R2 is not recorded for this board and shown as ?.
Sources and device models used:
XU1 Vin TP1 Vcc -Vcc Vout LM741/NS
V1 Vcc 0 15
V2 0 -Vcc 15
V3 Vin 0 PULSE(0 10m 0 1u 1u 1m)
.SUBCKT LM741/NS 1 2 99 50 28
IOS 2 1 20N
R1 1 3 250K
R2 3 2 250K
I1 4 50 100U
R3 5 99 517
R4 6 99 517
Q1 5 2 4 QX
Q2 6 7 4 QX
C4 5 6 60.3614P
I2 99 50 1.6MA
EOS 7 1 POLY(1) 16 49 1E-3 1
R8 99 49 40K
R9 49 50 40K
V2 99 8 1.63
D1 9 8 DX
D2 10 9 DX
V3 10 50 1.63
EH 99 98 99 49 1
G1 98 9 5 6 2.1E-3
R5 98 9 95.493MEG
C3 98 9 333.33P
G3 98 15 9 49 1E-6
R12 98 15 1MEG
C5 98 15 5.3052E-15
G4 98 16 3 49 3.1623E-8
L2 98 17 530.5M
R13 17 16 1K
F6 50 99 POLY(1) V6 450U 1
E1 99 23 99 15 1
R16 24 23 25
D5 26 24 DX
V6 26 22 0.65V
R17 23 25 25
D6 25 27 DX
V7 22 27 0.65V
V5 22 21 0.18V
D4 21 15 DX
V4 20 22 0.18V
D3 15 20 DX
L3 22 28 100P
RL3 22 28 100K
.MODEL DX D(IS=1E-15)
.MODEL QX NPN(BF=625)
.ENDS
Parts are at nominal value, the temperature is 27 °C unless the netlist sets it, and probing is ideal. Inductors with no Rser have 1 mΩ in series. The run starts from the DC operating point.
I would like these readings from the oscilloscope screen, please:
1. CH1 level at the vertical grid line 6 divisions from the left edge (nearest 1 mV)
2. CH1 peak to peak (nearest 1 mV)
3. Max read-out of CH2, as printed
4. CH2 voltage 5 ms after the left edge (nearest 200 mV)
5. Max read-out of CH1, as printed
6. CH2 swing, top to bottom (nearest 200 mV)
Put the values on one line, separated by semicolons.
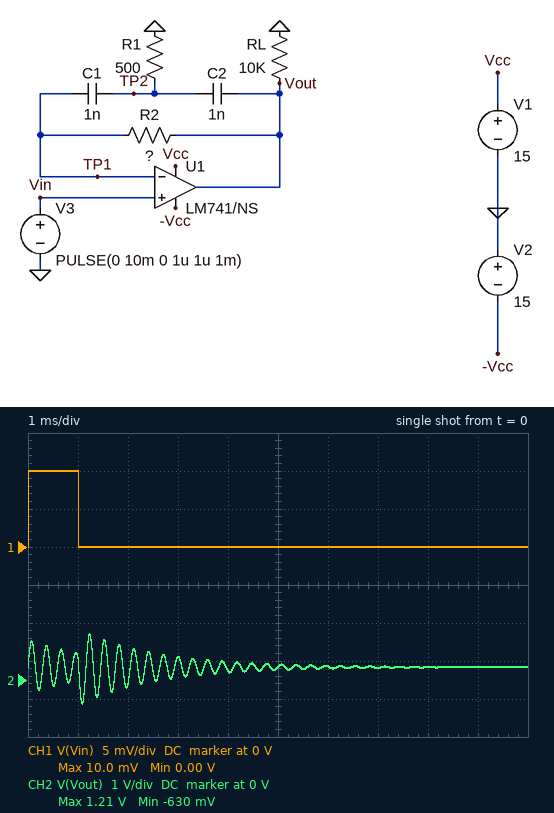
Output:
0 V; 10 mV; 1.21 V; 400 mV; 10.0 mV; 1.8 V
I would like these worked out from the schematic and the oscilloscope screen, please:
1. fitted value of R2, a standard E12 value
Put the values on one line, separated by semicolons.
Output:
3.3 MΩ
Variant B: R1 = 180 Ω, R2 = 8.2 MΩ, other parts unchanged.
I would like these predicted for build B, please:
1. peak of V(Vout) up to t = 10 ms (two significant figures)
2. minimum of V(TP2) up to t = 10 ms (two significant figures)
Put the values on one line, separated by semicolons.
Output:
2.3 V; -4.5 mV
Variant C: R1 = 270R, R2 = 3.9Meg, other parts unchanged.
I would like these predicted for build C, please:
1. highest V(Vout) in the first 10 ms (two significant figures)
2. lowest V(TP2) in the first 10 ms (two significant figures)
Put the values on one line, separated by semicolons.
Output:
1.3 V; -5.6 mV
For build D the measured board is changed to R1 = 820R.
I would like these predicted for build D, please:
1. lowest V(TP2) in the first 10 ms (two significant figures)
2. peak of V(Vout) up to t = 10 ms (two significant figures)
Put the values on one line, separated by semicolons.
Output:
-7.6 mV; 900 mV
